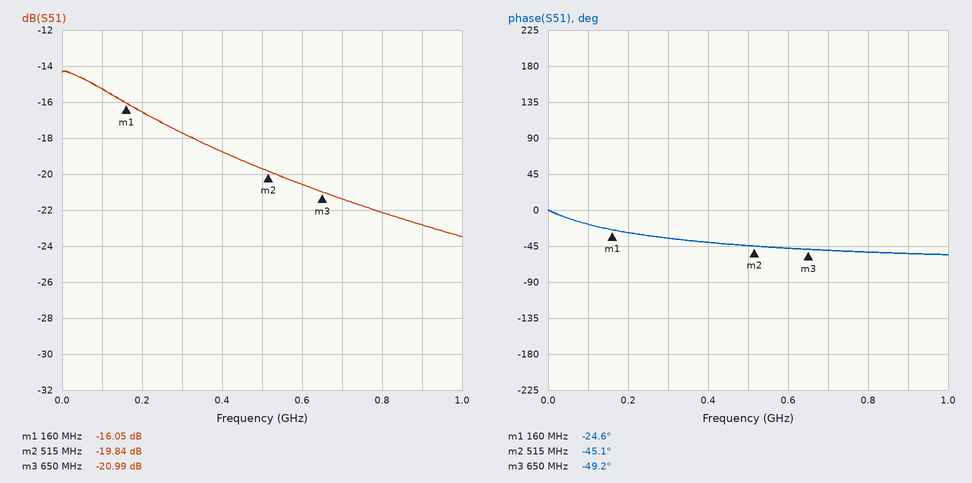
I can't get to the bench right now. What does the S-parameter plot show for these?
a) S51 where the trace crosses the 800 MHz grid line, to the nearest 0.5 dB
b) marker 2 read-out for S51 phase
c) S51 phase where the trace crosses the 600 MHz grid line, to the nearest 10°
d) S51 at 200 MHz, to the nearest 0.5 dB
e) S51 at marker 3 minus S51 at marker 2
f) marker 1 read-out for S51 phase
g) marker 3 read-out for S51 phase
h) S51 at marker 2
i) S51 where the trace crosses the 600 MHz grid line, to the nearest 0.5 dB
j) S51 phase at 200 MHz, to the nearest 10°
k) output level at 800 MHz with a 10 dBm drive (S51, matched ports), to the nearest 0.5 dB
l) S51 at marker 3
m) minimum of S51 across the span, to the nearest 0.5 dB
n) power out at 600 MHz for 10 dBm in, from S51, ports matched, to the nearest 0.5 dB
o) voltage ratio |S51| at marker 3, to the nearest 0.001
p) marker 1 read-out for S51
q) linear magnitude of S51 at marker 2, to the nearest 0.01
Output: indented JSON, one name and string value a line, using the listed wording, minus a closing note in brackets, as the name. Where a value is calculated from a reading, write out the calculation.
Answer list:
{
  "S51 where the trace crosses the 800 MHz grid line, to the nearest 0.5 dB": "-22.0 dB",
  "marker 2 read-out for S51 phase": "-45.1°",
  "S51 phase where the trace crosses the 600 MHz grid line, to the nearest 10°": "-50°",
  "S51 at 200 MHz, to the nearest 0.5 dB": "-16.5 dB",
  "S51 at marker 3 minus S51 at marker 2": "-20.99 − (-19.84) = -1.15 dB",
  "marker 1 read-out for S51 phase": "-24.6°",
  "marker 3 read-out for S51 phase": "-49.2°",
  "S51 at marker 2": "-19.84 dB",
  "S51 where the trace crosses the 600 MHz grid line, to the nearest 0.5 dB": "-20.5 dB",
  "S51 phase at 200 MHz, to the nearest 10°": "-30°",
  "output level at 800 MHz with a 10 dBm drive (S51, matched ports), to the nearest 0.5 dB": "10 dBm + (-22.0 dB) = -12.0 dBm",
  "S51 at marker 3": "-20.99 dB",
  "minimum of S51 across the span, to the nearest 0.5 dB": "-23.5 dB",
  "power out at 600 MHz for 10 dBm in, from S51, ports matched, to the nearest 0.5 dB": "10 dBm + (-20.5 dB) = -10.5 dBm",
  "voltage ratio |S51| at marker 3, to the nearest 0.001": "10^(-20.99/20) ≈ 0.089",
  "marker 1 read-out for S51": "-16.05 dB",
  "linear magnitude of S51 at marker 2, to the nearest 0.01": "10^(-19.84/20) ≈ 0.10"
}
